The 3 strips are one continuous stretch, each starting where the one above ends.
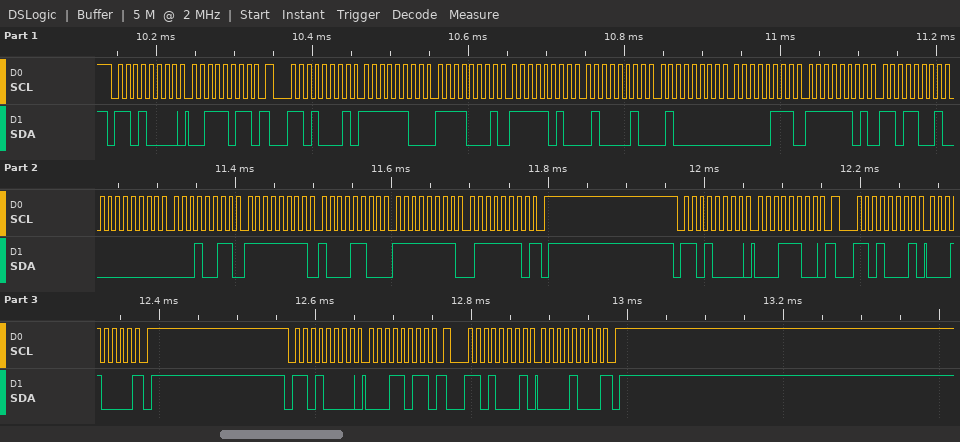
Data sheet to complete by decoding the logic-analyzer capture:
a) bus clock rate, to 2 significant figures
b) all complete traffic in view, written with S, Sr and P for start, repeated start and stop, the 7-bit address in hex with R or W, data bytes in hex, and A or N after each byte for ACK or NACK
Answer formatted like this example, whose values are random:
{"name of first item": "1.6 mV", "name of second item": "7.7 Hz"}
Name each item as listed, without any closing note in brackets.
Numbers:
{"bus clock rate, to 2 significant figures": "100 kHz", "all complete traffic in view, written with S, Sr and P for start, repeated start and stop, the 7-bit address in hex with R or W, data bytes in hex, and A or N after each byte for ACK or NACK": "S 68W A 3B A Sr 68R A FC A F1 A FA A 42 A 40 A 07 A FD A D9 A 00 A 13 A FF A 8C A FF A 7E N P S 68W A 1C A Sr 68R A 10 N P S 68W A 1B A Sr 68R A 08 N P"}
